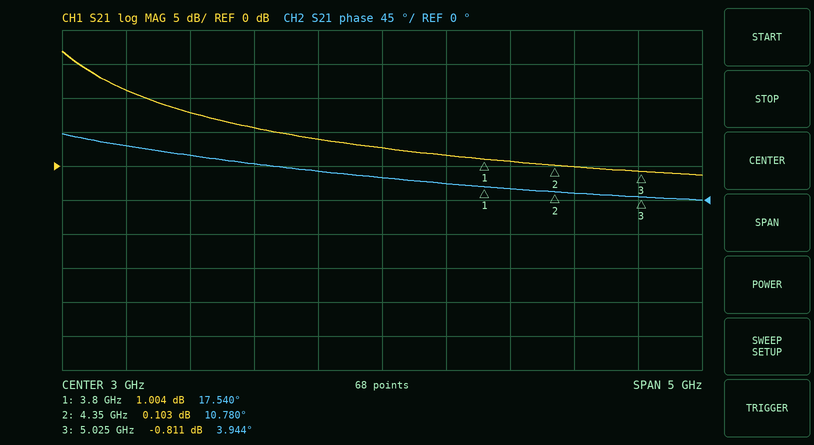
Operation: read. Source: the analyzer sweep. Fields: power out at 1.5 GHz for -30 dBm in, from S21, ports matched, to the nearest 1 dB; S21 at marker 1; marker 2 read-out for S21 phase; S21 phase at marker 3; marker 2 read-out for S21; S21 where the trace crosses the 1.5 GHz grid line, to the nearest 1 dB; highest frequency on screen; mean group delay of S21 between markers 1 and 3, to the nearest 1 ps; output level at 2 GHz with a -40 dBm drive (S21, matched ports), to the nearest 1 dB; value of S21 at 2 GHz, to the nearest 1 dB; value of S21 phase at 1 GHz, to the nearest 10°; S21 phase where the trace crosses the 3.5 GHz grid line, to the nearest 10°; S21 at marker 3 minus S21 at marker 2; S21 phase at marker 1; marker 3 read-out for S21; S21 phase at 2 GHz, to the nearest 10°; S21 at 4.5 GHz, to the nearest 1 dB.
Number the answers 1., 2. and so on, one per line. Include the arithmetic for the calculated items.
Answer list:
1. -30 dBm + (8 dB) = -22 dBm
2. 1.004 dB
3. 10.780°
4. 3.944°
5. 0.103 dB
6. 8 dB
7. 5.5 GHz
8. −(3.944° − (17.54°))/(360° × 1.225 GHz) ≈ 31 ps
9. -40 dBm + (6 dB) = -34 dBm
10. 6 dB
11. 70°
12. 20°
13. -0.811 − (0.103) = -0.914 dB
14. 17.540°
15. -0.811 dB
16. 50°
17. 0 dB
